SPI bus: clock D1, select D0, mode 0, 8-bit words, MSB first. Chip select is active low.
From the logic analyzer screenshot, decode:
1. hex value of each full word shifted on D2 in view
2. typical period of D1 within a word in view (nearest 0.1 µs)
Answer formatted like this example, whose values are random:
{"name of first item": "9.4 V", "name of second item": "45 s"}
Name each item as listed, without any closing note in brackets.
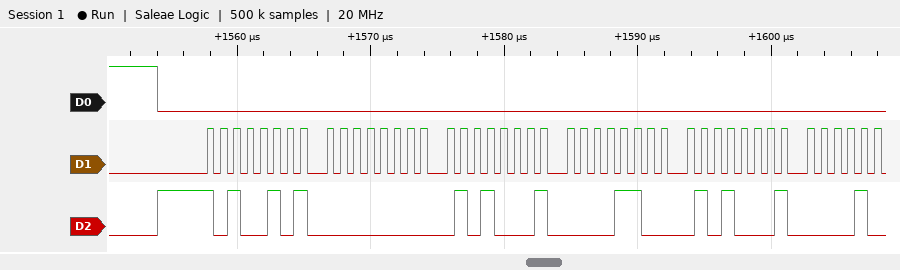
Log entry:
{"hex value of each full word shifted on D2 in view": "A5, 00, 51, 0C, 51", "typical period of D1 within a word in view": "1 µs"}
